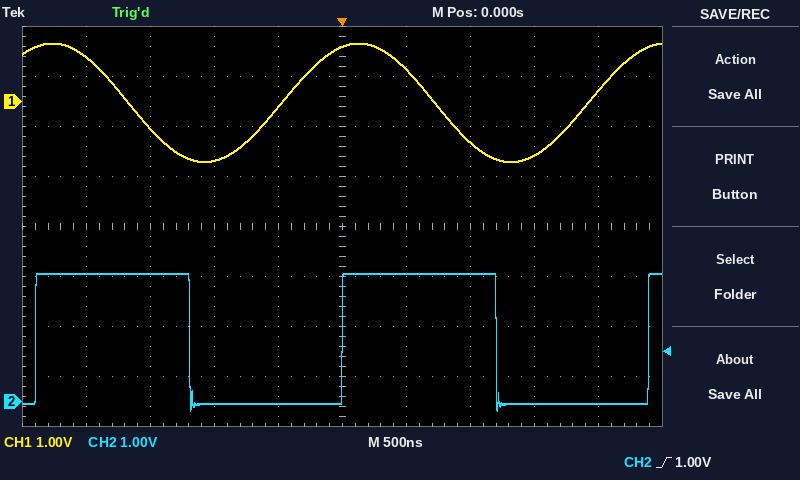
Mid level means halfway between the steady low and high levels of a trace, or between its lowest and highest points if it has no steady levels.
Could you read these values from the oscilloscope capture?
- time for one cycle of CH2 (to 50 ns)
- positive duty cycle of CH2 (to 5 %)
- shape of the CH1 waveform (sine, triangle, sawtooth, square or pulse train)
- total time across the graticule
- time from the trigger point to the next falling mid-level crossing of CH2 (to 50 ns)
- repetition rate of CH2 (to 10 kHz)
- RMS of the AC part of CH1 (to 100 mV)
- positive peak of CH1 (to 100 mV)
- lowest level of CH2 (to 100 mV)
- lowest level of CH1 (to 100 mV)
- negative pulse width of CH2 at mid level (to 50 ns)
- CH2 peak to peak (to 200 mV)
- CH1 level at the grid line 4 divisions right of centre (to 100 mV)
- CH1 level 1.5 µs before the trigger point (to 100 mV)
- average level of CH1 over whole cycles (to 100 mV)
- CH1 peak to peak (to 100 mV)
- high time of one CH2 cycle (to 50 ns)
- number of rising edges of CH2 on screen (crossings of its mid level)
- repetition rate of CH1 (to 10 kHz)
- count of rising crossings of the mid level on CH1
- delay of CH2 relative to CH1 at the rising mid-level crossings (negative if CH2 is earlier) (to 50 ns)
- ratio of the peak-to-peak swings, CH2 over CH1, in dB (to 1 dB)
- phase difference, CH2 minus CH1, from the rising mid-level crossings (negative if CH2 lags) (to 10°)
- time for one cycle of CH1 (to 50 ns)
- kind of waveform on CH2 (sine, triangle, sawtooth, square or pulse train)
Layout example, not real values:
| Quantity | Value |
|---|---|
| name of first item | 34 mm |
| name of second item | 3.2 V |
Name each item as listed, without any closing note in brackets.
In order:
| Quantity | Value |
|---|---|
| time for one cycle of CH2 | 2.40 µs |
| positive duty cycle of CH2 | 50 % |
| shape of the CH1 waveform | sine |
| total time across the graticule | 5 µs |
| time from the trigger point to the next falling mid-level crossing of CH2 | 1.20 µs |
| repetition rate of CH2 | 420 kHz |
| RMS of the AC part of CH1 | 800 mV |
| positive peak of CH1 | 1.2 V |
| lowest level of CH2 | -200 mV |
| lowest level of CH1 | -1.2 V |
| negative pulse width of CH2 at mid level | 1.20 µs |
| CH2 peak to peak | 2.8 V |
| CH1 level at the grid line 4 divisions right of centre | 200 mV |
| CH1 level 1.5 µs before the trigger point | -500 mV |
| average level of CH1 over whole cycles | 0.0 V |
| CH1 peak to peak | 2.4 V |
| high time of one CH2 cycle | 1.20 µs |
| number of rising edges of CH2 on screen | 3 |
| repetition rate of CH1 | 420 kHz |
| count of rising crossings of the mid level on CH1 | 2 |
| delay of CH2 relative to CH1 at the rising mid-level crossings (negative if CH2 is earlier) | +450 ns |
| ratio of the peak-to-peak swings, CH2 over CH1, in dB | 1 dB |
| phase difference, CH2 minus CH1, from the rising mid-level crossings (negative if CH2 lags) | -70° |
| time for one cycle of CH1 | 2.40 µs |
| kind of waveform on CH2 | square |
